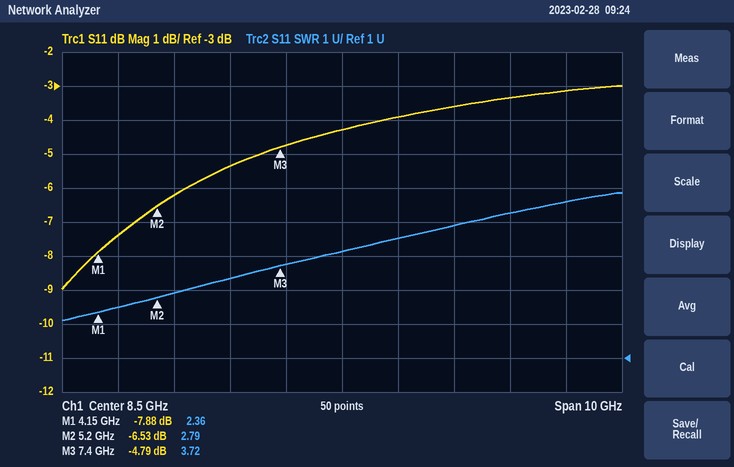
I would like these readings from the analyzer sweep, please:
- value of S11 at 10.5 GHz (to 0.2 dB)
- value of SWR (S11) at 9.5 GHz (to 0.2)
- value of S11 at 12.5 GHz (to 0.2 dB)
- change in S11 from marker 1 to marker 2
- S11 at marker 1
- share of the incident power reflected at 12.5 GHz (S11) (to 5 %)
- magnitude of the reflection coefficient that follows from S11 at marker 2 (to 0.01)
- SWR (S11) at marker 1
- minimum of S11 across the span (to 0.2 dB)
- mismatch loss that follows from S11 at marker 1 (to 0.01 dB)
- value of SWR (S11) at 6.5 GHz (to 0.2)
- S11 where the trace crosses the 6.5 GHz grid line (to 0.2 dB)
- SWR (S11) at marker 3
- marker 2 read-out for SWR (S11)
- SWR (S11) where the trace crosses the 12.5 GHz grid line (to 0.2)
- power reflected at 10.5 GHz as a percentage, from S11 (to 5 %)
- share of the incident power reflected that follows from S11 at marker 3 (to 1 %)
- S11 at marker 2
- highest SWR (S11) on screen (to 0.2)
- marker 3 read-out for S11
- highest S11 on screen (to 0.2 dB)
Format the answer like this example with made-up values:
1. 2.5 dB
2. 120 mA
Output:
1. -3.6 dB
2. 4.6
3. -3.2 dB
4. 1.35 dB
5. -7.88 dB
6. 50 %
7. 0.47
8. 2.36
9. -9.0 dB
10. 0.77 dB
11. 3.4
12. -5.4 dB
13. 3.72
14. 2.79
15. 5.6
16. 45 %
17. 33 %
18. -6.53 dB
19. 5.8
20. -4.79 dB
21. -3.0 dB
